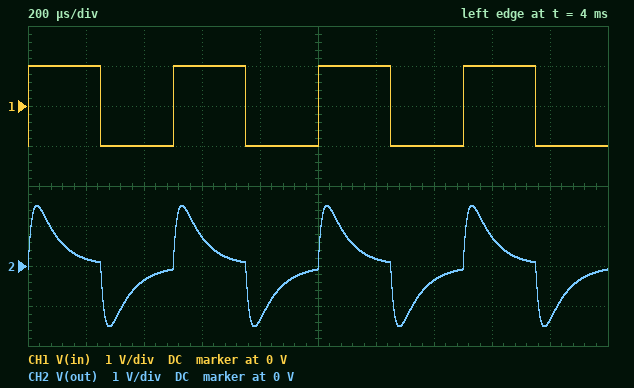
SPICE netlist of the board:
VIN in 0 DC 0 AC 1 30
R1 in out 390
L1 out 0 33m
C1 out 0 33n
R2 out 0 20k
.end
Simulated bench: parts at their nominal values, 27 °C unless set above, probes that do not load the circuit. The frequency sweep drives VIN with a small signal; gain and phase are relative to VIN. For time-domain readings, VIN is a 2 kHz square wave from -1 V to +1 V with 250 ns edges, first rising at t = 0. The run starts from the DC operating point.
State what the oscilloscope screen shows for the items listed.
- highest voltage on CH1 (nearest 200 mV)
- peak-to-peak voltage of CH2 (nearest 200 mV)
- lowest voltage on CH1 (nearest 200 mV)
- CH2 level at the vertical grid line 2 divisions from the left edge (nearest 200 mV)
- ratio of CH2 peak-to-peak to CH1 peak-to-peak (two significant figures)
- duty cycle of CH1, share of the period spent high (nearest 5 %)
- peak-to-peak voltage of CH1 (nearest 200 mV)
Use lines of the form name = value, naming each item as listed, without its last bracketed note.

highest voltage on CH1 = 1.0 V
peak-to-peak voltage of CH2 = 3.0 V
lowest voltage on CH1 = -1.0 V
CH2 level at the vertical grid line 2 divisions from the left edge = -400 mV
ratio of CH2 peak-to-peak to CH1 peak-to-peak = 1.5
duty cycle of CH1, share of the period spent high = 50 %
peak-to-peak voltage of CH1 = 2.0 V
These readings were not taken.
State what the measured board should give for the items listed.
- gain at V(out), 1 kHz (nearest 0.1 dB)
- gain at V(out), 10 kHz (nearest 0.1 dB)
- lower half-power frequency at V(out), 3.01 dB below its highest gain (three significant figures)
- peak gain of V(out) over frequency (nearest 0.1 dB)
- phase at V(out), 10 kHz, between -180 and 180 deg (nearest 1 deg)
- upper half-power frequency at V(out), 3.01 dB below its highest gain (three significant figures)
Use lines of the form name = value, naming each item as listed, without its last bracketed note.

gain at V(out), 1 kHz = -6.3 dB
gain at V(out), 10 kHz = -1.5 dB
lower half-power frequency at V(out), 3.01 dB below its highest gain = 1.63 kHz
peak gain of V(out) over frequency = -0.2 dB
phase at V(out), 10 kHz, between -180 and 180 deg = -31 deg
upper half-power frequency at V(out), 3.01 dB below its highest gain = 14.2 kHz
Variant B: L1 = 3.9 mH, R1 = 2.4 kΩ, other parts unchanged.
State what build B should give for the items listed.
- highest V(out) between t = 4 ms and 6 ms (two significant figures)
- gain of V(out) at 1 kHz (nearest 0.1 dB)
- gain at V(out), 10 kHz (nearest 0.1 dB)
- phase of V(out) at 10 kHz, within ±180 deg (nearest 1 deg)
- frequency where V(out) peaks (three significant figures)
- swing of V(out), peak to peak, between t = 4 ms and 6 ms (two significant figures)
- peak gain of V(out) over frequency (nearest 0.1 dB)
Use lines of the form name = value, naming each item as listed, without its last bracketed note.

highest V(out) between t = 4 ms and 6 ms = 310 mV
gain of V(out) at 1 kHz = -39.8 dB
gain at V(out), 10 kHz = -13.9 dB
phase of V(out) at 10 kHz, within ±180 deg = 77 deg
frequency where V(out) peaks = 14.0 kHz
swing of V(out), peak to peak, between t = 4 ms and 6 ms = 610 mV
peak gain of V(out) over frequency = -1.0 dB
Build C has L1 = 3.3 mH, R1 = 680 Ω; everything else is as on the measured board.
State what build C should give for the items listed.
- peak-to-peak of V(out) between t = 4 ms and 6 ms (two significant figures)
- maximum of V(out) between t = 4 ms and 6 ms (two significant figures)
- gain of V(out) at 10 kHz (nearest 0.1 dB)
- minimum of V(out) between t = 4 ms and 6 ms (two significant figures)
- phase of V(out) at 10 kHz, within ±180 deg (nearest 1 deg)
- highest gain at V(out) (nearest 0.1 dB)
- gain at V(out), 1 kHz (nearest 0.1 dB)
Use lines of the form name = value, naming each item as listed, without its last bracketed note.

peak-to-peak of V(out) between t = 4 ms and 6 ms = 1.3 V
maximum of V(out) between t = 4 ms and 6 ms = 670 mV
gain of V(out) at 10 kHz = -6.6 dB
minimum of V(out) between t = 4 ms and 6 ms = -670 mV
phase of V(out) at 10 kHz, within ±180 deg = 61 deg
highest gain at V(out) = -0.3 dB
gain at V(out), 1 kHz = -30.3 dB
